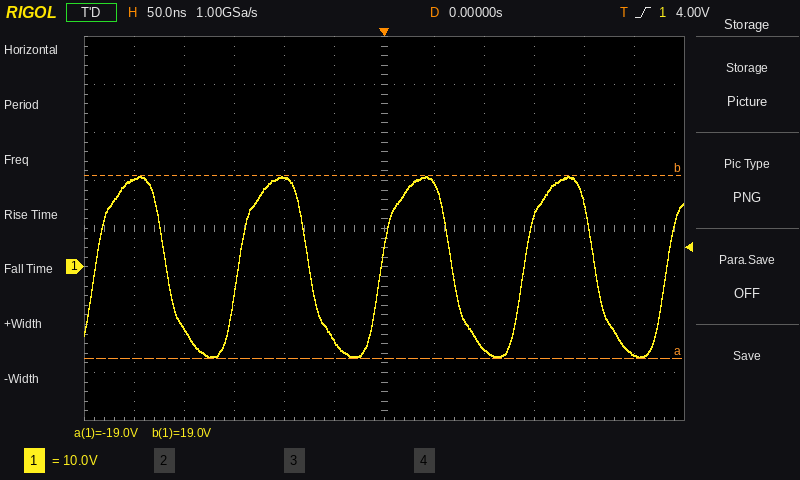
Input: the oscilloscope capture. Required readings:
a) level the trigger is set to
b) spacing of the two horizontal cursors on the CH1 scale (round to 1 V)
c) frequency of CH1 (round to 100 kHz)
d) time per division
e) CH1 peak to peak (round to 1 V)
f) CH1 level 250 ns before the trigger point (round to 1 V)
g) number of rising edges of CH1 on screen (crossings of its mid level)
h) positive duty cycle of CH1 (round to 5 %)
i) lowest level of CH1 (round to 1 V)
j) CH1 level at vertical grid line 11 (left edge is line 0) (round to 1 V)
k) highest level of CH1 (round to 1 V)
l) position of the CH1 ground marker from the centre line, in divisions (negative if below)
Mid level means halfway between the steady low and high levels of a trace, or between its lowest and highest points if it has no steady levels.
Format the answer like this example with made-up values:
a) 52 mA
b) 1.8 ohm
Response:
a) 4.00 V
b) 38 V
c) 7.0 MHz
d) 50 ns
e) 38 V
f) 18 V
g) 5
h) 50 %
i) -19 V
j) -18 V
k) 19 V
l) -0.8 div
